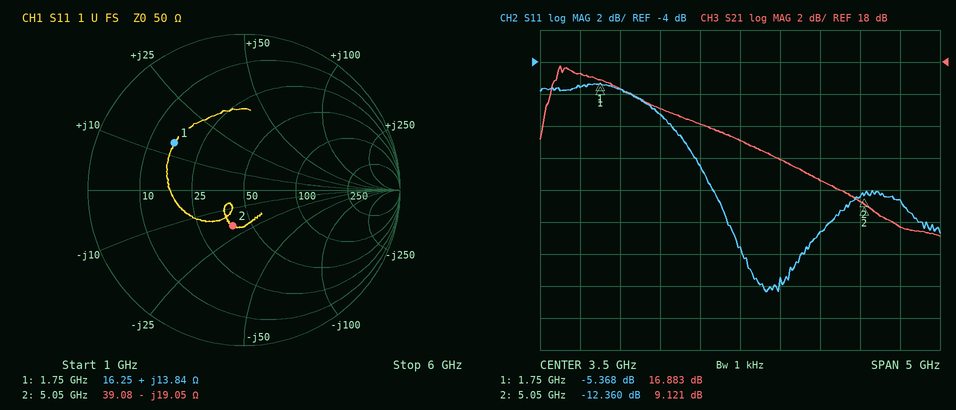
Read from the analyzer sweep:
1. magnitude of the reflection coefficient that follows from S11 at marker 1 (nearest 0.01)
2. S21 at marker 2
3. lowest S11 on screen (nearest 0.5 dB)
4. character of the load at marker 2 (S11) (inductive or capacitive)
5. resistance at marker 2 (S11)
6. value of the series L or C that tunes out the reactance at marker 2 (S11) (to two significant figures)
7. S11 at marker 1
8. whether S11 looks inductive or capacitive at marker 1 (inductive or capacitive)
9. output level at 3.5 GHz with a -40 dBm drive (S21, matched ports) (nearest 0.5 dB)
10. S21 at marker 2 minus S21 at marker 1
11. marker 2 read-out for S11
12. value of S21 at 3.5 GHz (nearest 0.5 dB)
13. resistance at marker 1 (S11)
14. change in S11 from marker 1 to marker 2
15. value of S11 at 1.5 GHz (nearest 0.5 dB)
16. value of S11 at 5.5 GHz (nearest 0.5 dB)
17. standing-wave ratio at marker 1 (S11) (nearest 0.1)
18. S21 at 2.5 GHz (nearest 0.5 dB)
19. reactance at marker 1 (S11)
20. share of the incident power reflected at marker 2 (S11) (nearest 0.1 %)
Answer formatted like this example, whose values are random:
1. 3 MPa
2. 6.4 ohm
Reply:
1. 0.54
2. 9.121 dB
3. -18.5 dB
4. capacitive
5. 39.08 Ω
6. 600 pH
7. -5.368 dB
8. inductive
9. -27.0 dBm
10. -7.762 dB
11. -12.360 dB
12. 13.0 dB
13. 16.25 Ω
14. -6.992 dB
15. -5.5 dB
16. -12.5 dB
17. 3.3
18. 15.0 dB
19. +13.84 Ω
20. 5.8 %
